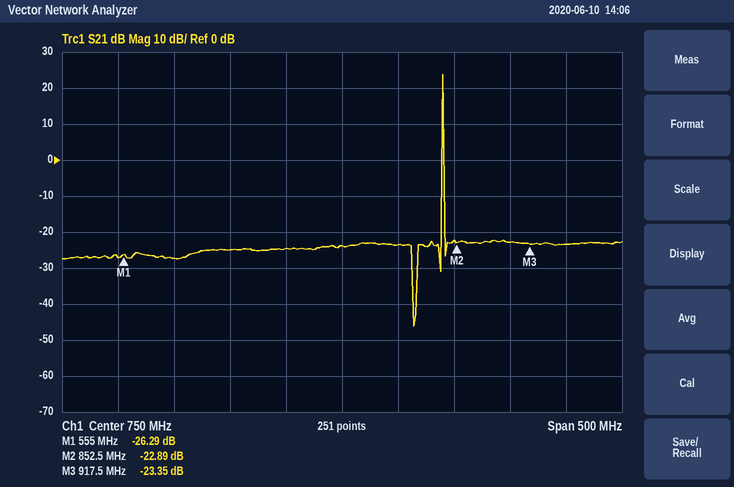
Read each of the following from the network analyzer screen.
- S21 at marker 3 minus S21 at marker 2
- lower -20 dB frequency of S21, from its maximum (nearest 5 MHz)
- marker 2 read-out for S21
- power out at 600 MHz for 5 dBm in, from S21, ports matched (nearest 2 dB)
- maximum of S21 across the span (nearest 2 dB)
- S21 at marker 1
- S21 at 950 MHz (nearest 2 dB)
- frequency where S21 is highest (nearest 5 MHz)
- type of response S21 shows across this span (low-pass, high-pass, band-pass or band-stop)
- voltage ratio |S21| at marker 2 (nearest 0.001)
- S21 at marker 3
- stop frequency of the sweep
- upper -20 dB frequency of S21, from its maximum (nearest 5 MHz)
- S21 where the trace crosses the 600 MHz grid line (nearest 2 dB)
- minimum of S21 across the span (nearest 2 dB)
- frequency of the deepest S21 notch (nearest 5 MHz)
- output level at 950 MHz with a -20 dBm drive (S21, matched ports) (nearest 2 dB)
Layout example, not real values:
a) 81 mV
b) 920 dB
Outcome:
a) -0.46 dB
b) 840 MHz
c) -22.89 dB
d) -22 dBm
e) 24 dB
f) -26.29 dB
g) -24 dB
h) 840 MHz
i) band-pass
j) 0.072
k) -23.35 dB
l) 1 GHz
m) 840 MHz
n) -28 dB
o) -46 dB
p) 815 MHz
q) -44 dBm
